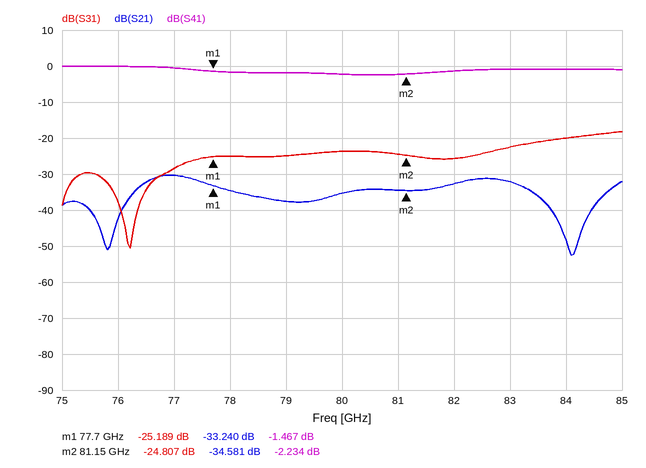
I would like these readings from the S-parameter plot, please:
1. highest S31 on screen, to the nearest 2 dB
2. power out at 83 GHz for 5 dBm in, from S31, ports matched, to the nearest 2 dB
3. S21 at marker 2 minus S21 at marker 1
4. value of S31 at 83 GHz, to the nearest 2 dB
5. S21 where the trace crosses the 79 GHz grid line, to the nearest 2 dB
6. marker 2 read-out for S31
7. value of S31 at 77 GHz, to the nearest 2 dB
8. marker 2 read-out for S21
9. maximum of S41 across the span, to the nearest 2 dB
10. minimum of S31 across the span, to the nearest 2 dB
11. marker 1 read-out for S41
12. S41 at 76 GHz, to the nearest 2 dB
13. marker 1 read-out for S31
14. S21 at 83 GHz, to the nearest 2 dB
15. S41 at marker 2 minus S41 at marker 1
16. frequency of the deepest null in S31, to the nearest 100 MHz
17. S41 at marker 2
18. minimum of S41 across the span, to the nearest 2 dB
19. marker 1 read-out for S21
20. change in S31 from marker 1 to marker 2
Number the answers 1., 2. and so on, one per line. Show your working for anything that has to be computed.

1. -18 dB
2. 5 dBm + (-22 dB) = -18 dBm
3. -34.581 − (-33.24) = -1.341 dB
4. -22 dB
5. -38 dB
6. -24.807 dB
7. -28 dB
8. -34.581 dB
9. 0 dB
10. -50 dB
11. -1.467 dB
12. 0 dB
13. -25.189 dB
14. -32 dB
15. -2.234 − (-1.467) = -0.767 dB
16. 76.2 GHz
17. -2.234 dB
18. -2 dB
19. -33.240 dB
20. -24.807 − (-25.189) = 0.382 dB
